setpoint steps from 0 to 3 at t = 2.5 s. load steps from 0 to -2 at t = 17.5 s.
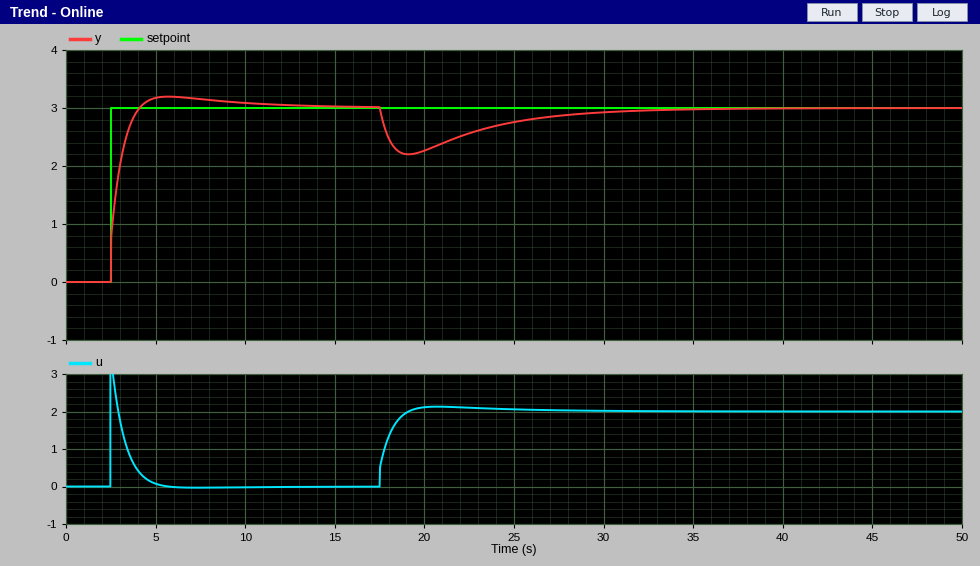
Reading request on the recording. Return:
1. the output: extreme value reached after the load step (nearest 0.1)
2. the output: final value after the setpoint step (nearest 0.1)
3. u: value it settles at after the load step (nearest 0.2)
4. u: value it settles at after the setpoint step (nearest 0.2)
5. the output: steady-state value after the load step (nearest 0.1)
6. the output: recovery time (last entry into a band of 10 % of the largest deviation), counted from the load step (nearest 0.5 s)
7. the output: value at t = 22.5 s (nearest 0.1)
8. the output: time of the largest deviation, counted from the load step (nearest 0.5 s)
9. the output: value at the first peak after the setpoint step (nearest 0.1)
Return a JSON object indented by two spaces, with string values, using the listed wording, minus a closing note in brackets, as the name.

{
  "the output: extreme value reached after the load step": "2.2",
  "the output: final value after the setpoint step": "3.0",
  "u: value it settles at after the load step": "2.0",
  "u: value it settles at after the setpoint step": "0.0",
  "the output: steady-state value after the load step": "3.0",
  "the output: recovery time (last entry into a band of 10 % of the largest deviation), counted from the load step": "12.0 s",
  "the output: value at t = 22.5 s": "2.6",
  "the output: time of the largest deviation, counted from the load step": "1.5 s",
  "the output: value at the first peak after the setpoint step": "3.2"
}
